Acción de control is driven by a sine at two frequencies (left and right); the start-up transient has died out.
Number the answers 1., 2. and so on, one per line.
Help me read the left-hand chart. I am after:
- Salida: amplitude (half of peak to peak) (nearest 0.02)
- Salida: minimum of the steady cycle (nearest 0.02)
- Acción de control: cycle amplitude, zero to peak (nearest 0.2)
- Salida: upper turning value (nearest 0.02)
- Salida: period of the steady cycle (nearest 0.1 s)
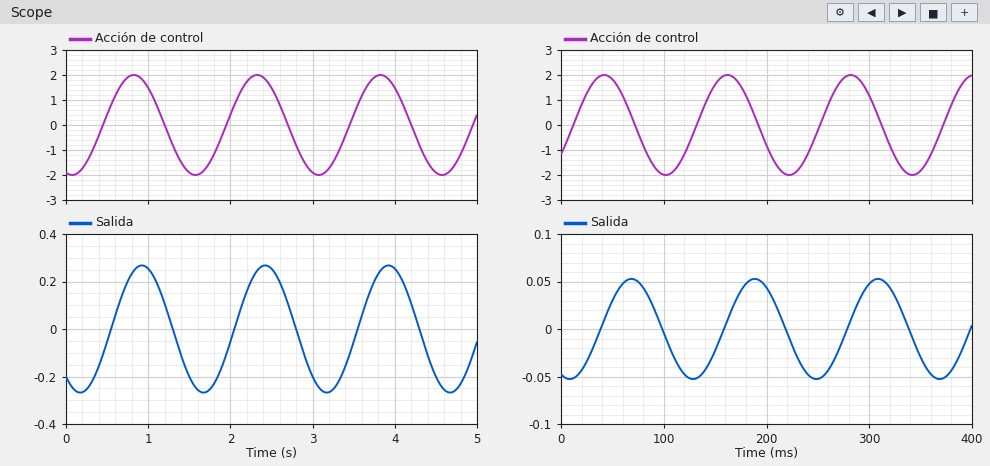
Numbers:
1. 0.26
2. -0.26
3. 2.0
4. 0.26
5. 1.5 s
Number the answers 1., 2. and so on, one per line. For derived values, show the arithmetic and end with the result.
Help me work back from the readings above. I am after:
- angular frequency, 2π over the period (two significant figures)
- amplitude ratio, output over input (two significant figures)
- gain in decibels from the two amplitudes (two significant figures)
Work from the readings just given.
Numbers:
1. 2π / 1.5 = 4.2 rad/s
2. 0.26 / 2 = 0.13
3. 20 log10(0.26 / 2) = -18 dB
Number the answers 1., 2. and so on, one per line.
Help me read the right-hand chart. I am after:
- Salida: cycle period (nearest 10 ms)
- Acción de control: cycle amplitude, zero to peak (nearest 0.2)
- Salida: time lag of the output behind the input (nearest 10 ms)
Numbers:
1. 120 ms
2. 2.0
3. 30 ms
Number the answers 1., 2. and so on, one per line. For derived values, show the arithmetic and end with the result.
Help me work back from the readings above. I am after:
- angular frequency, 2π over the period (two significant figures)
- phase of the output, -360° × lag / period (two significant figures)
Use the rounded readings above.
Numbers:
1. 2π / 120 = 0.052 rad/ms
2. -360 × 30 / 120 = -90°
